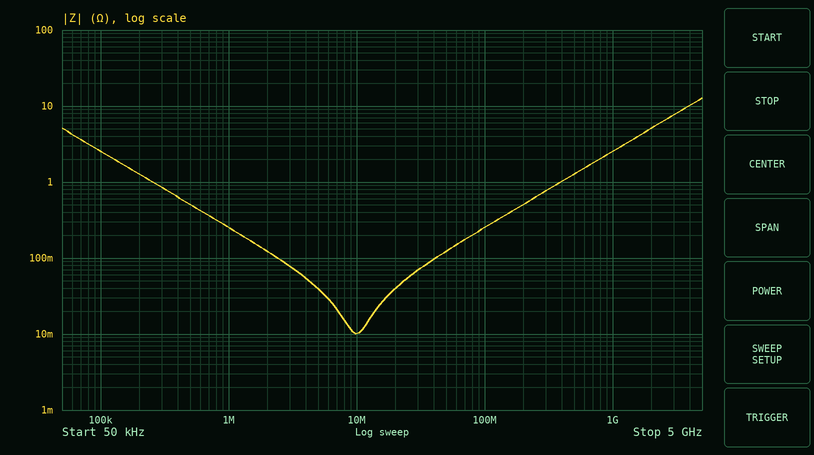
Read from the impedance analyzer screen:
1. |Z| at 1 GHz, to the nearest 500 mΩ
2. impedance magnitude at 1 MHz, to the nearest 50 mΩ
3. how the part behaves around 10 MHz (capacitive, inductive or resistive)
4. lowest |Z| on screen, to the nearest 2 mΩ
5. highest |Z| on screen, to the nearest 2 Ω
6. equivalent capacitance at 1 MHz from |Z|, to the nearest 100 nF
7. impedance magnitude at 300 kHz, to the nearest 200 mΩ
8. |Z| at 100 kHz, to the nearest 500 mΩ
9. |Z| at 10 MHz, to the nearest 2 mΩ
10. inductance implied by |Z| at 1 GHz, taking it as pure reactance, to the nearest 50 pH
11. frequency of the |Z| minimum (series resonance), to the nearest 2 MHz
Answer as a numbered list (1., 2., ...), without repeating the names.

1. 2.5 Ω
2. 250 mΩ
3. resistive
4. 10 mΩ
5. 12 Ω
6. 600 nF
7. 800 mΩ
8. 2.5 Ω
9. 10 mΩ
10. 400 pH
11. 10 MHz
